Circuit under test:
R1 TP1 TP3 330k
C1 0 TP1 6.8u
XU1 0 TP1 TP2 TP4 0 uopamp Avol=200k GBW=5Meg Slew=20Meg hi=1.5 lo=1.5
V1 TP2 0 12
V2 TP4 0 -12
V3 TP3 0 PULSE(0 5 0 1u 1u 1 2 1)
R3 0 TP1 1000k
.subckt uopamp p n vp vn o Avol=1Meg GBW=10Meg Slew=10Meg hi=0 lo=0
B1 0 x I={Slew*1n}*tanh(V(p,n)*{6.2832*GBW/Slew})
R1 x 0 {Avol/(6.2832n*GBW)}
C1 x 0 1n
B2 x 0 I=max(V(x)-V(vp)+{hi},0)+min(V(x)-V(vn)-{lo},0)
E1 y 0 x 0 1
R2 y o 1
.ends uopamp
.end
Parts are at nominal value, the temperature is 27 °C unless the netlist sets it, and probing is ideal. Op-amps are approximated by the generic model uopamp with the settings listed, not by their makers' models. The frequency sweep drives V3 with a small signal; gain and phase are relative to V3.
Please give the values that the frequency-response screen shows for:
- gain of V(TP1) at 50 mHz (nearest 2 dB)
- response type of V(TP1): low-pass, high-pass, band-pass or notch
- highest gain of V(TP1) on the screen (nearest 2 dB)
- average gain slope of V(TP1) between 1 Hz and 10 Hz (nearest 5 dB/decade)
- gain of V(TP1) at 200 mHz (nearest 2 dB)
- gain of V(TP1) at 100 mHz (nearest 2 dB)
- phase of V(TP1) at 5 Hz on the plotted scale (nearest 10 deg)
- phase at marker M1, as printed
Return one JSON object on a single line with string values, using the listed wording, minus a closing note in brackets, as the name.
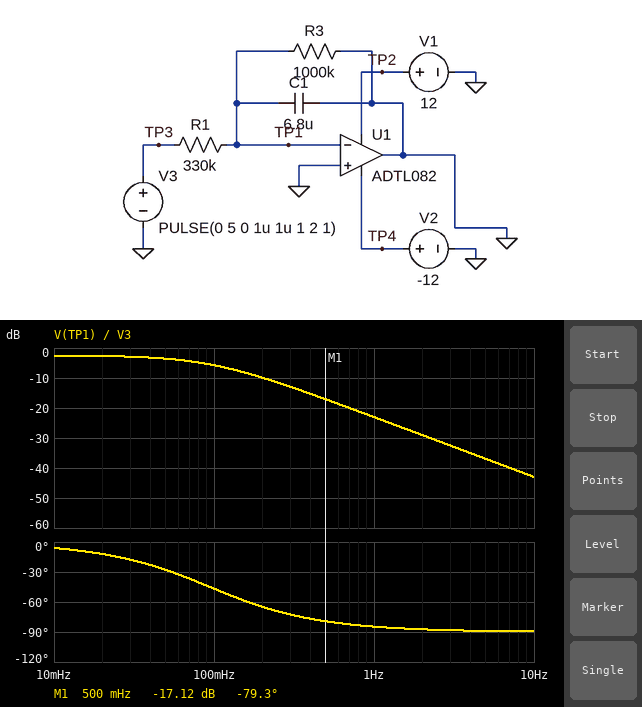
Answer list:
{"gain of V(TP1) at 50 mHz": "-4 dB", "response type of V(TP1): low-pass, high-pass, band-pass or notch": "low-pass", "highest gain of V(TP1) on the screen": "-2 dB", "average gain slope of V(TP1) between 1 Hz and 10 Hz": "-20 dB/decade", "gain of V(TP1) at 200 mHz": "-10 dB", "gain of V(TP1) at 100 mHz": "-6 dB", "phase of V(TP1) at 5 Hz on the plotted scale": "-90 deg", "phase at marker M1, as printed": "-79.3 deg"}
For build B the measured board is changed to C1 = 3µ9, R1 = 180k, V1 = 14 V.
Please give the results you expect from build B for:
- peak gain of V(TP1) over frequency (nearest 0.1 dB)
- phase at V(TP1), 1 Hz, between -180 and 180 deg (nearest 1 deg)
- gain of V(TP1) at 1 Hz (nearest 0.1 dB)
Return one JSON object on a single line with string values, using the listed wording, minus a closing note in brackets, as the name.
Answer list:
{"peak gain of V(TP1) over frequency": "-1.4 dB", "phase at V(TP1), 1 Hz, between -180 and 180 deg": "-75 deg", "gain of V(TP1) at 1 Hz": "-13.2 dB"}
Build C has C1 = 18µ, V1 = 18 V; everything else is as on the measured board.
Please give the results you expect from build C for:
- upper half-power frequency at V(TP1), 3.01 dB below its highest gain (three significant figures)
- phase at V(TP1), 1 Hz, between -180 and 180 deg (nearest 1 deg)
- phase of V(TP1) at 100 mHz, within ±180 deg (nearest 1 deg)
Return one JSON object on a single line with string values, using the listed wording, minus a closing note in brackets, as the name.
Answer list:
{"upper half-power frequency at V(TP1), 3.01 dB below its highest gain": "35.6 mHz", "phase at V(TP1), 1 Hz, between -180 and 180 deg": "-88 deg", "phase of V(TP1) at 100 mHz, within ±180 deg": "-70 deg"}
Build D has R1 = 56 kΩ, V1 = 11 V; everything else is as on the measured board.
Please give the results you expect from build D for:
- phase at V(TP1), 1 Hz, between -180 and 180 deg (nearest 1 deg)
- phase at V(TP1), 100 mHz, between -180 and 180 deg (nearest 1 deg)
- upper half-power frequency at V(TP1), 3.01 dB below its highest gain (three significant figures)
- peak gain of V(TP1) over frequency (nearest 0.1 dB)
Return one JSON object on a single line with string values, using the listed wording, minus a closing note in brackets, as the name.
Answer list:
{"phase at V(TP1), 1 Hz, between -180 and 180 deg": "-66 deg", "phase at V(TP1), 100 mHz, between -180 and 180 deg": "-13 deg", "upper half-power frequency at V(TP1), 3.01 dB below its highest gain": "441 mHz", "peak gain of V(TP1) over frequency": "-0.5 dB"}
